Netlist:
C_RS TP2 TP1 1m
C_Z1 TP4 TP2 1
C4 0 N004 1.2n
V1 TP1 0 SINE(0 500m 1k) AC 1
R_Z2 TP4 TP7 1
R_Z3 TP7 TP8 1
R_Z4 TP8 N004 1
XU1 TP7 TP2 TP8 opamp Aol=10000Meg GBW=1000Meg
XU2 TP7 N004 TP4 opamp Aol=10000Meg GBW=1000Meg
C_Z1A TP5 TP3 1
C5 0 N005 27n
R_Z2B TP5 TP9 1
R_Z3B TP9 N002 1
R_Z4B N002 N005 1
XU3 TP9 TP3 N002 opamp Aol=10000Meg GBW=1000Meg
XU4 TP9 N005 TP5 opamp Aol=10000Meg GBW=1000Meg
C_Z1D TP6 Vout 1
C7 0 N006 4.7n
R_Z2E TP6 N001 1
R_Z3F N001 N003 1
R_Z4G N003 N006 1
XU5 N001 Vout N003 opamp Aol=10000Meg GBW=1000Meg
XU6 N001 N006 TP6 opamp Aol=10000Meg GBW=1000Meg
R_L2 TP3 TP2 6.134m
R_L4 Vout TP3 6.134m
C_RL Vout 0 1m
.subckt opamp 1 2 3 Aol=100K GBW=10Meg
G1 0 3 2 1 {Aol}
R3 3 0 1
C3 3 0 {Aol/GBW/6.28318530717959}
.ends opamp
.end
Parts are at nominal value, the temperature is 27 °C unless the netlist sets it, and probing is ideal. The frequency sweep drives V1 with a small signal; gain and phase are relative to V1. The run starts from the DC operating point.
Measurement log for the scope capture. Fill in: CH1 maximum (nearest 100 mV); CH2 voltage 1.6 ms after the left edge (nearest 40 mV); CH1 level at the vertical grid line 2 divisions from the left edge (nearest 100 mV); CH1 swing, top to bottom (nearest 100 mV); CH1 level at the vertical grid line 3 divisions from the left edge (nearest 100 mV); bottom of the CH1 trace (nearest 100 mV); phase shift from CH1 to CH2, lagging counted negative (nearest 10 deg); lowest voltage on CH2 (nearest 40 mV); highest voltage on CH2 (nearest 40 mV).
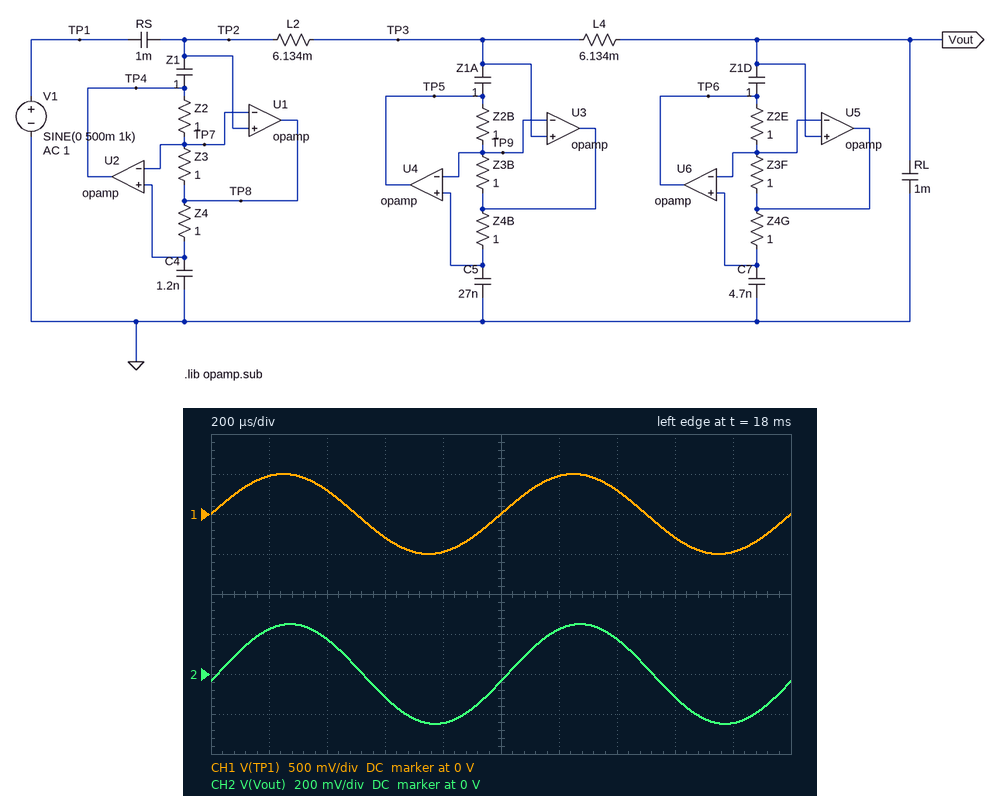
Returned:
500 mV
-120 mV
300 mV
1.0 V
-300 mV
-500 mV
-10 deg
-240 mV
240 mV
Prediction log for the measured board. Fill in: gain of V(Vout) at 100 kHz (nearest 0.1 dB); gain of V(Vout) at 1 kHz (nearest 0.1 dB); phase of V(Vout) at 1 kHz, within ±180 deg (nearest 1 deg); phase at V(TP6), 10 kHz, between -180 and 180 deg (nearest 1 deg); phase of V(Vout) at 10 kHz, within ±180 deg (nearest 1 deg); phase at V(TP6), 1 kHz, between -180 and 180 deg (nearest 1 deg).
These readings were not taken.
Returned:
-59.3 dB
-6.0 dB
-8 deg
-79 deg
-79 deg
-8 deg
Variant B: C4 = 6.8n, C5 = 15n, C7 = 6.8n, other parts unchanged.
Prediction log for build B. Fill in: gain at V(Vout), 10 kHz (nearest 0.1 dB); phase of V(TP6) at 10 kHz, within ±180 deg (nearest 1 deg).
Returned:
-6.6 dB
-71 deg
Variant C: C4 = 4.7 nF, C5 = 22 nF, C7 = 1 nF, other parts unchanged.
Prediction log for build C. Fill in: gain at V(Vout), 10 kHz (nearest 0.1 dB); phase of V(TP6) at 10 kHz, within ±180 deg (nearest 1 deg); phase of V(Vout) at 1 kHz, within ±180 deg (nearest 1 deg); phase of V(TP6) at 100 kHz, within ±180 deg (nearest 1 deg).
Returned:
-7.0 dB
-72 deg
-7 deg
-10 deg
